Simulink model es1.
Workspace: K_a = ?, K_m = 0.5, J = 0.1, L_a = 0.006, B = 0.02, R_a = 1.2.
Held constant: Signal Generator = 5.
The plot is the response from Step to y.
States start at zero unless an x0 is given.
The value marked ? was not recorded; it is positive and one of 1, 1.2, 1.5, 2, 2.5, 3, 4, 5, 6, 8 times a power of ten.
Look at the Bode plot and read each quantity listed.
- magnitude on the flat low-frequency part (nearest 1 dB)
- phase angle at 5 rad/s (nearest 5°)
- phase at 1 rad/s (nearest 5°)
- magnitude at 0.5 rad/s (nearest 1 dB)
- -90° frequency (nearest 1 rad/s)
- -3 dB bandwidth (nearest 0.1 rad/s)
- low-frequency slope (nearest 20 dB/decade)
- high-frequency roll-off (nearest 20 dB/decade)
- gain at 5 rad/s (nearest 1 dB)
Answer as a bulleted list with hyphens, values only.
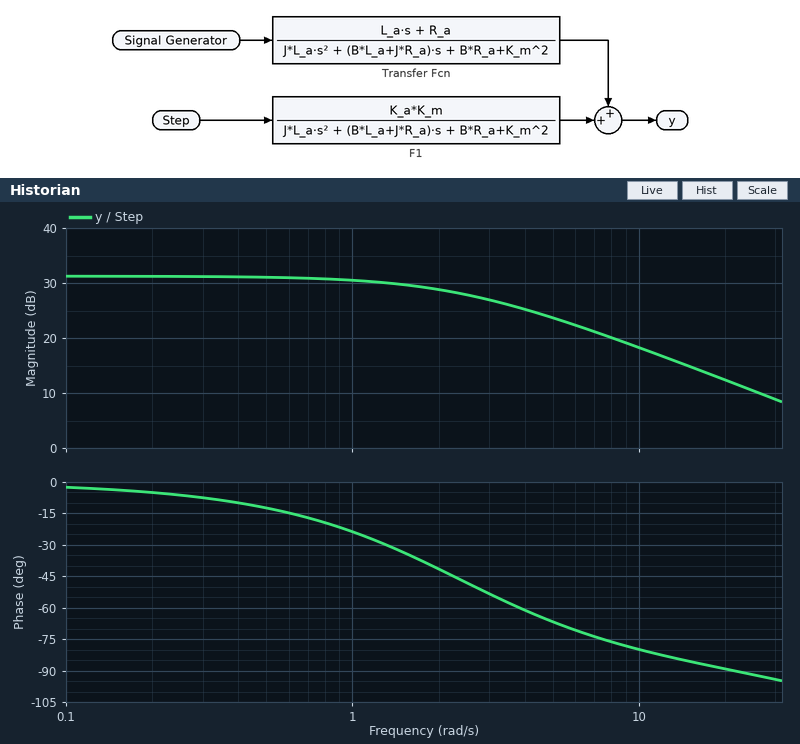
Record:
- 31 dB
- -65°
- -25°
- 31 dB
- 21 rad/s
- 2.3 rad/s
- 0 dB/decade
- -20 dB/decade
- 24 dB
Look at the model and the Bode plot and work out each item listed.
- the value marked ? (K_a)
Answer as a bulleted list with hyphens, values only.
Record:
- 20
